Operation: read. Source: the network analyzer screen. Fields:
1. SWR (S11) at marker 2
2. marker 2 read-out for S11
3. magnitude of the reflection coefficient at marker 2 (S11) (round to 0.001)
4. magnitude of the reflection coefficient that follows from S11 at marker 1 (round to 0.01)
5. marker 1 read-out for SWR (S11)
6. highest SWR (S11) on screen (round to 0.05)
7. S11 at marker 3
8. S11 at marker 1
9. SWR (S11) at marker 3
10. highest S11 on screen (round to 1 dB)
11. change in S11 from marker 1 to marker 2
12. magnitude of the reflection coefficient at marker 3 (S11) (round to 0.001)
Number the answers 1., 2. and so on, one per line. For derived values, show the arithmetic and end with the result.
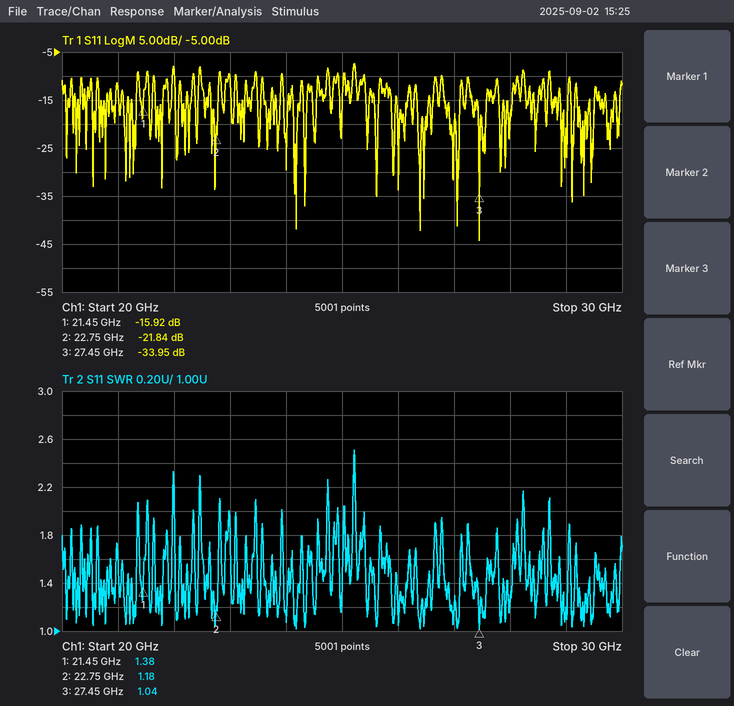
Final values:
1. 1.18
2. -21.84 dB
3. 10^(-21.84/20) ≈ 0.081
4. 10^(-15.92/20) ≈ 0.16
5. 1.38
6. 2.50
7. -33.95 dB
8. -15.92 dB
9. 1.04
10. -7 dB
11. -21.84 − (-15.92) = -5.92 dB
12. 10^(-33.95/20) ≈ 0.020
